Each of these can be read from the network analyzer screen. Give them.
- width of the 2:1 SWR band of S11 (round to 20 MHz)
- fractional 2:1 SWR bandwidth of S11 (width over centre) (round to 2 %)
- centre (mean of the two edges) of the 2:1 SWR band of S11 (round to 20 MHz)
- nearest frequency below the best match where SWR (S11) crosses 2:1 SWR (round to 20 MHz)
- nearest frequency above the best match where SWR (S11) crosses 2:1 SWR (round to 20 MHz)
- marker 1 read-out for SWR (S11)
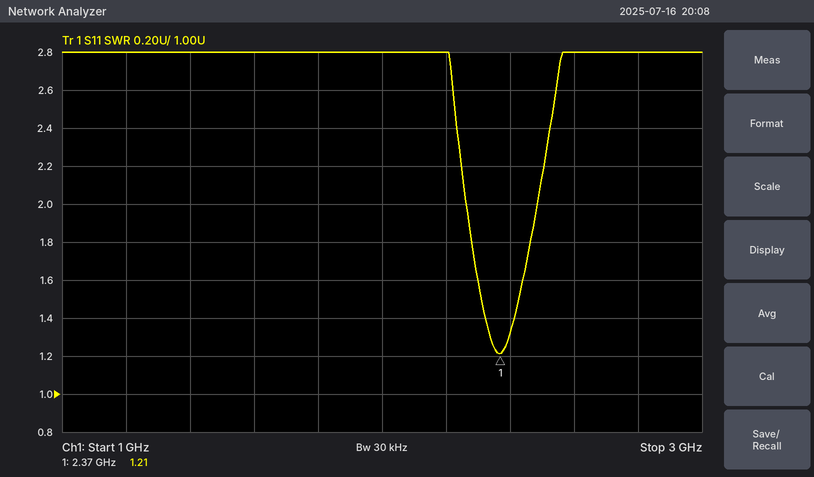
220 MHz
10 %
2.38 GHz
2.26 GHz
2.48 GHz
1.21
